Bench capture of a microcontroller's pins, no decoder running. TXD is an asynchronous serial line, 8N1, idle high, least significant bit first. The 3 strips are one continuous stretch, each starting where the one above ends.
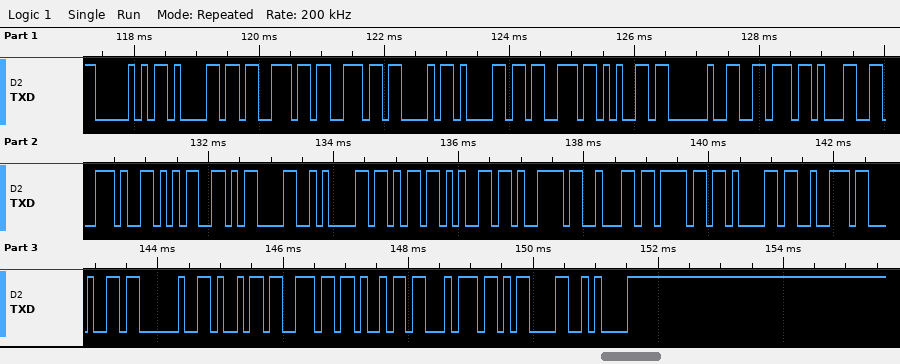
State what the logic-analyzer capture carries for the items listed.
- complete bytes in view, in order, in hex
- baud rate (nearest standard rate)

0x50 0x61 0x73 0x73 0x43 0x61 0x73 0x65 0x20 0x76 0x31 0x2E 0x35 0x0D 0x0A 0x6B 0x65 0x79 0x62 0x6F 0x61 0x72 0x64 0x20 0x69 0x6E 0x69 0x74 0x0D 0x0A
9600 baud
